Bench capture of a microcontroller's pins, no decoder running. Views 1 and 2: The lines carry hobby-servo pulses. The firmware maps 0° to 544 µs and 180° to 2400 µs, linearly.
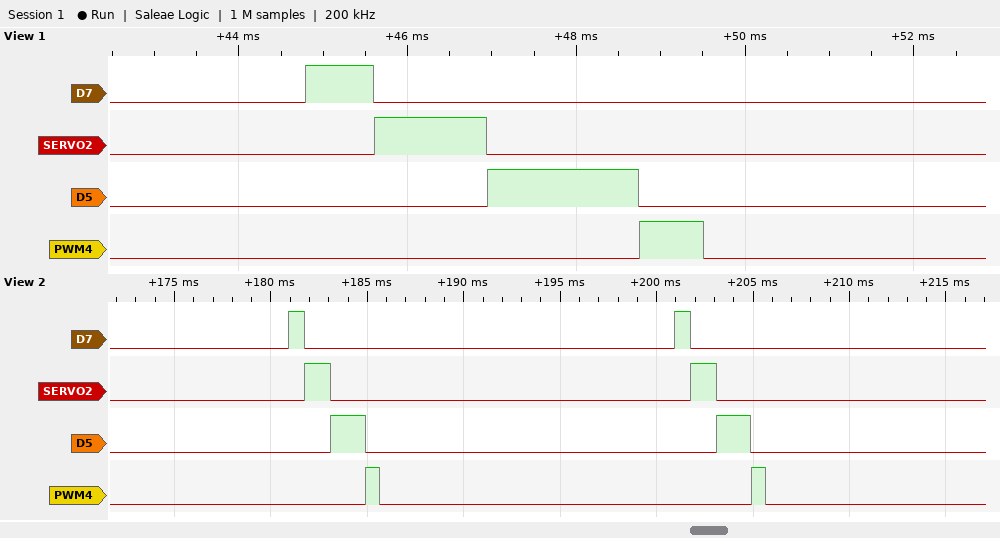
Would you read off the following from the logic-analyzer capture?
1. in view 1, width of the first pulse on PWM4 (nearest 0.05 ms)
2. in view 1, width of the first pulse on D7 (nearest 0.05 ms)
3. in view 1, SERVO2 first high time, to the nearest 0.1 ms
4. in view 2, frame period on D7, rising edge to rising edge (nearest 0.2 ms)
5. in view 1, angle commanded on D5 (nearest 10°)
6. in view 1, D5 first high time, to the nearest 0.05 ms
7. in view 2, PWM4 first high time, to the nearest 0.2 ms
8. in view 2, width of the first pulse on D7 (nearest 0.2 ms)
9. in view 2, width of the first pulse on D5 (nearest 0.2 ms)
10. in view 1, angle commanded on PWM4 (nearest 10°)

0.75 ms
0.80 ms
1.3 ms
20.0 ms
120°
1.80 ms
0.8 ms
0.8 ms
1.8 ms
20°
